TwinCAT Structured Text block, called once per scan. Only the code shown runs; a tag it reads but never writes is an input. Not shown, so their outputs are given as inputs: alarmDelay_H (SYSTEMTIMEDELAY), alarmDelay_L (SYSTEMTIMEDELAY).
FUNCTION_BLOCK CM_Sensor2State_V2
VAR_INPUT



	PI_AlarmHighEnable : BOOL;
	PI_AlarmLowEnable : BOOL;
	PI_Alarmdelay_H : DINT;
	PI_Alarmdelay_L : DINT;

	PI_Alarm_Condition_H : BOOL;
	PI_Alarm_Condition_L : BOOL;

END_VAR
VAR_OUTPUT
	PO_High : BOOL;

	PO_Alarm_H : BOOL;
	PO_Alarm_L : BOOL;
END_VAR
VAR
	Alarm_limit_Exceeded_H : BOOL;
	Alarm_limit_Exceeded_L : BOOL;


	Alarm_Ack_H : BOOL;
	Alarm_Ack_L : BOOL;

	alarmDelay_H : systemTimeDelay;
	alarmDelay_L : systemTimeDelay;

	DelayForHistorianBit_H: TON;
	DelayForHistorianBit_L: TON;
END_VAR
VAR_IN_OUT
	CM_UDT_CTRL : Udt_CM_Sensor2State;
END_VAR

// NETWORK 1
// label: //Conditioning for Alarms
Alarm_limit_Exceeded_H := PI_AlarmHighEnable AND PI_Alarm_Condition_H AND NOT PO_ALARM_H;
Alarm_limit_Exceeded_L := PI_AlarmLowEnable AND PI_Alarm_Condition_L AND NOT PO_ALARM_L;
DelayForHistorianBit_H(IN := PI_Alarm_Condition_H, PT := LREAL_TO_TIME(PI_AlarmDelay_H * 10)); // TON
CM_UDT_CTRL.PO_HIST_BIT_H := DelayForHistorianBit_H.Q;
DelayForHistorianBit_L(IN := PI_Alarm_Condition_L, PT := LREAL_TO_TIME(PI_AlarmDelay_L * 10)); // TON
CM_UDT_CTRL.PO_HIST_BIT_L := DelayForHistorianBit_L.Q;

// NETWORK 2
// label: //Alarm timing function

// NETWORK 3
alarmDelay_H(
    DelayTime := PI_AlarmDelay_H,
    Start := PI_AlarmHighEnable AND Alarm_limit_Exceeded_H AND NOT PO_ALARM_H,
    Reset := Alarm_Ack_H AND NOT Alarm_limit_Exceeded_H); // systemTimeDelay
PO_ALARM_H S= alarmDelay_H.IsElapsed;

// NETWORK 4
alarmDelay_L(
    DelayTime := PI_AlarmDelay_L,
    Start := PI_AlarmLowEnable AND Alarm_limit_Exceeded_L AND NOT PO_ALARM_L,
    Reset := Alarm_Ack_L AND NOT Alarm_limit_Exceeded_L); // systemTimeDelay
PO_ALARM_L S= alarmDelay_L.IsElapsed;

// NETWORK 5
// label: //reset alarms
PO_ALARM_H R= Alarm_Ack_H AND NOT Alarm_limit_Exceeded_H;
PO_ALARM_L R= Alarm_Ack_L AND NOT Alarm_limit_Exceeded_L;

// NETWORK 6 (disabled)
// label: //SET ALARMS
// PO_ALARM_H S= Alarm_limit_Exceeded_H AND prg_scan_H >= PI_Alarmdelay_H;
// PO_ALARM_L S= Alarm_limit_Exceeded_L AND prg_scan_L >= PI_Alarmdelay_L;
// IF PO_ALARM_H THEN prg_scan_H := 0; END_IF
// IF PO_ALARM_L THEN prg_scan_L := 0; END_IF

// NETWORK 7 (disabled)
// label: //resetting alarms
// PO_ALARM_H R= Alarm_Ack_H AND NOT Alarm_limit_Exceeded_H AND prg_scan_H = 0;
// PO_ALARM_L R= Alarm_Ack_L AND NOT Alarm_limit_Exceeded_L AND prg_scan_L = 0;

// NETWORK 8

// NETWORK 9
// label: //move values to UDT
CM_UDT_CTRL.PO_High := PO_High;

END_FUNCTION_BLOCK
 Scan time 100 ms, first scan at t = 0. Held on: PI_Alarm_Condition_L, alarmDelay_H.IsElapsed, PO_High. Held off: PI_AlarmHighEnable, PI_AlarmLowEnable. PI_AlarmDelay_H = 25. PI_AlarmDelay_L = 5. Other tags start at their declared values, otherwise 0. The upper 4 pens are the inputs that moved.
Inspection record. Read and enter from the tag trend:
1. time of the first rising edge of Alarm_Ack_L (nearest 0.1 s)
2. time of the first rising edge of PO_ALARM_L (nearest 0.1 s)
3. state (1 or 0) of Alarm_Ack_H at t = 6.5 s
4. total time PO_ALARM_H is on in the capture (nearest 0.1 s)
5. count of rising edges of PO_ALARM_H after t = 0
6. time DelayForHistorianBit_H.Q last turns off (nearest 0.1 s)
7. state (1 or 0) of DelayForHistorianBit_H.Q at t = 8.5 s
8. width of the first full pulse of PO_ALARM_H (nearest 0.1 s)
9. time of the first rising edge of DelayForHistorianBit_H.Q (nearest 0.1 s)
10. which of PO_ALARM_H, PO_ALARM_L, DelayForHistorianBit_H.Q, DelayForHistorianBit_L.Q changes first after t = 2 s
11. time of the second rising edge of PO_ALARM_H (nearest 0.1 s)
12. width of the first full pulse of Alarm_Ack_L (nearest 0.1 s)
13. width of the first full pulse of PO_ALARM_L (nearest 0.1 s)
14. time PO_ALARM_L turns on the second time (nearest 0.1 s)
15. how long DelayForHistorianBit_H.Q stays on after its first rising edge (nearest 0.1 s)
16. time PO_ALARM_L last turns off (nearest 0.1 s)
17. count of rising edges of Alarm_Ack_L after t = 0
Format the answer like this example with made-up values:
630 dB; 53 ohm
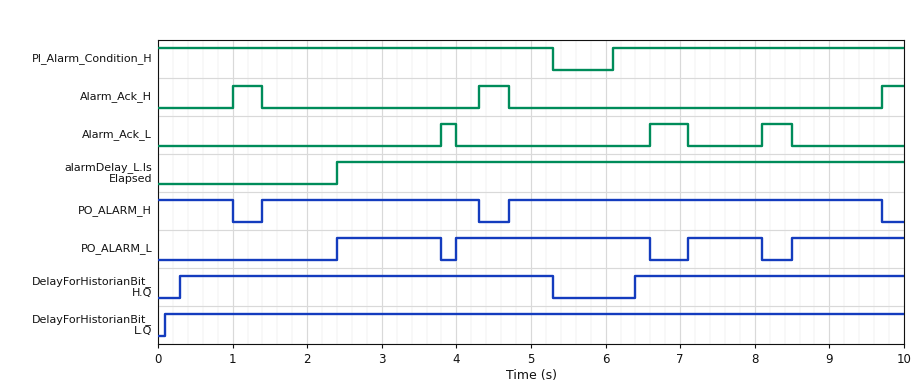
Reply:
3.8 s; 2.4 s; 0; 8.9 s; 2; 5.3 s; 1; 2.9 s; 0.3 s; PO_ALARM_L; 4.7 s; 0.2 s; 1.4 s; 4.0 s; 5.0 s; 8.1 s; 3
